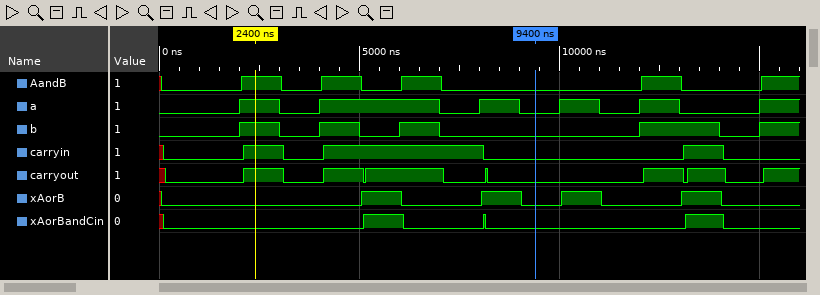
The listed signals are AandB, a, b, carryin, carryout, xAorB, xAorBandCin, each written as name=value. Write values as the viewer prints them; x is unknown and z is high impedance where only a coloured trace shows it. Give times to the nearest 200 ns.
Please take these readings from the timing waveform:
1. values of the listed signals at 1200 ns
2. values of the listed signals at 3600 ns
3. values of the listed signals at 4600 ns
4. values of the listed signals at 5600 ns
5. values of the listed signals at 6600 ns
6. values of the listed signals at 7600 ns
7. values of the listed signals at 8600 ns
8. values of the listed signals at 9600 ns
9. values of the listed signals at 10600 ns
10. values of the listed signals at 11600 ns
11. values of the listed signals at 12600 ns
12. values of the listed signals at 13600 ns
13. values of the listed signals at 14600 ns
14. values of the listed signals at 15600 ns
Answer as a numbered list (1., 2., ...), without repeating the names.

1. AandB=0, a=0, b=0, carryin=0, carryout=0, xAorB=0, xAorBandCin=0
2. AandB=0, a=0, b=0, carryin=0, carryout=0, xAorB=0, xAorBandCin=0
3. AandB=1, a=1, b=1, carryin=1, carryout=1, xAorB=0, xAorBandCin=0
4. AandB=0, a=1, b=0, carryin=1, carryout=1, xAorB=1, xAorBandCin=1
5. AandB=1, a=1, b=1, carryin=1, carryout=1, xAorB=0, xAorBandCin=0
6. AandB=0, a=0, b=0, carryin=1, carryout=0, xAorB=0, xAorBandCin=0
7. AandB=0, a=1, b=0, carryin=0, carryout=0, xAorB=1, xAorBandCin=0
8. AandB=0, a=0, b=0, carryin=0, carryout=0, xAorB=0, xAorBandCin=0
9. AandB=0, a=1, b=0, carryin=0, carryout=0, xAorB=1, xAorBandCin=0
10. AandB=0, a=0, b=0, carryin=0, carryout=0, xAorB=0, xAorBandCin=0
11. AandB=1, a=1, b=1, carryin=0, carryout=1, xAorB=0, xAorBandCin=0
12. AandB=0, a=0, b=1, carryin=1, carryout=1, xAorB=1, xAorBandCin=1
13. AandB=0, a=0, b=0, carryin=0, carryout=0, xAorB=0, xAorBandCin=0
14. AandB=1, a=1, b=1, carryin=0, carryout=1, xAorB=0, xAorBandCin=0
